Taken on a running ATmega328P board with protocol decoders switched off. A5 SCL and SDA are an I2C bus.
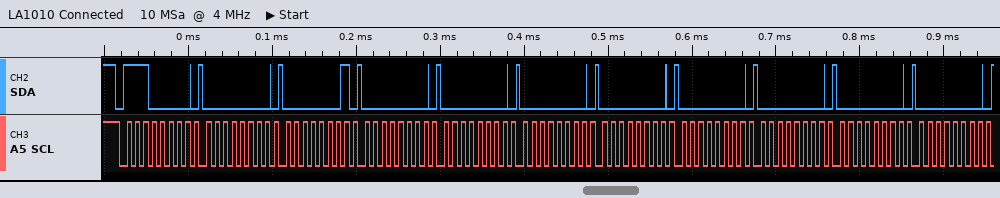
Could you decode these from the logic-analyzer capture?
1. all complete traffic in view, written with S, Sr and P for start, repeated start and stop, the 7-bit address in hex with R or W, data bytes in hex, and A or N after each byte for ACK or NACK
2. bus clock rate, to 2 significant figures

S 70W A 00 A 01 A 00 A 00 A 00 A 00 A 00 A 00 A 00 A 00 A
100 kHz
